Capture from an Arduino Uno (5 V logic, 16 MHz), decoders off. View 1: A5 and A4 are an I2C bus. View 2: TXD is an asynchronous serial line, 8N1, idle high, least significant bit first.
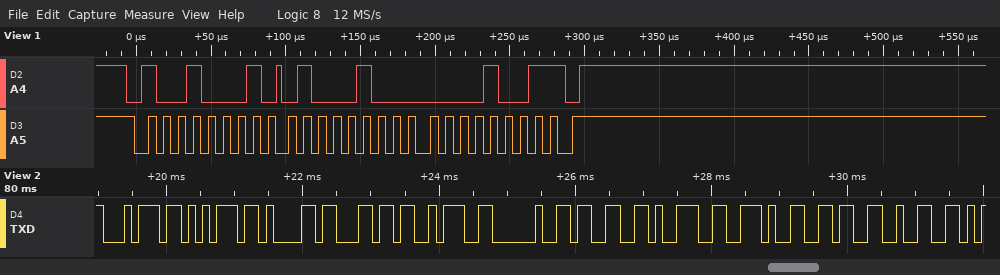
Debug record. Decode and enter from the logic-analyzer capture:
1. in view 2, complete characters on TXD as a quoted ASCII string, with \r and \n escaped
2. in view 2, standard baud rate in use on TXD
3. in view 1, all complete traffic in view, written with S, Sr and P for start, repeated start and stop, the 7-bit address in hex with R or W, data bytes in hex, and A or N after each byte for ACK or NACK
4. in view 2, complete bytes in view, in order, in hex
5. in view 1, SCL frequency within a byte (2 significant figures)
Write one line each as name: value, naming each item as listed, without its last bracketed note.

in view 2, complete characters on TXD as a quoted ASCII string, with \r and \n escaped: "tual: 39.62"
in view 2, standard baud rate in use on TXD: 9600 baud
in view 1, all complete traffic in view, written with S, Sr and P for start, repeated start and stop, the 7-bit address in hex with R or W, data bytes in hex, and A or N after each byte for ACK or NACK: S 48R A 44 A 09 N P
in view 2, complete bytes in view, in order, in hex: 74 75 61 6C 3A 20 33 39 2E 36 32
in view 1, SCL frequency within a byte: 100 kHz
